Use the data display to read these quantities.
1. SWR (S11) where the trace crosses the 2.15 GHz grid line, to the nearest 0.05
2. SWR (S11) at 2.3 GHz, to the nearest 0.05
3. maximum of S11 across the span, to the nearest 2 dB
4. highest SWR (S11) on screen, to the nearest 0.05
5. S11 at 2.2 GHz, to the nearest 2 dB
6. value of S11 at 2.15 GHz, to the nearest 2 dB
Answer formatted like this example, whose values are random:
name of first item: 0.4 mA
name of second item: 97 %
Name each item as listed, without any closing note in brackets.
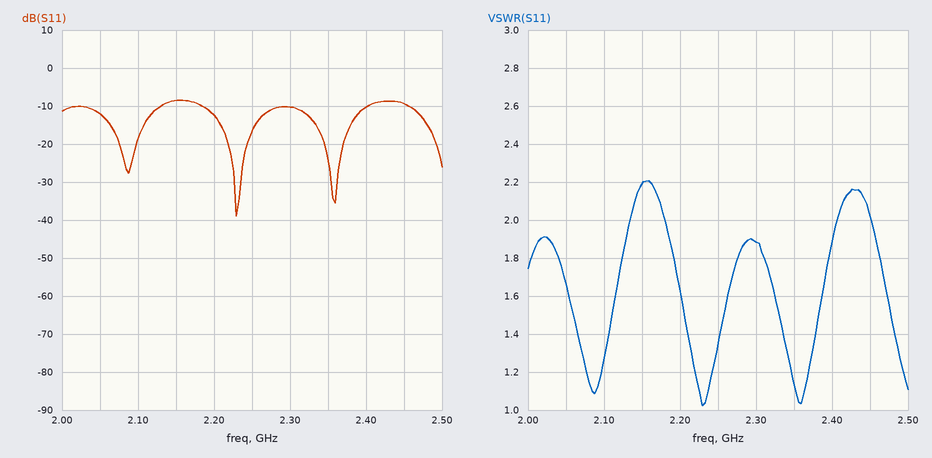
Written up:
SWR (S11) where the trace crosses the 2.15 GHz grid line, to the nearest 0.05: 2.20
SWR (S11) at 2.3 GHz, to the nearest 0.05: 1.90
maximum of S11 across the span, to the nearest 2 dB: -8 dB
highest SWR (S11) on screen, to the nearest 0.05: 2.20
S11 at 2.2 GHz, to the nearest 2 dB: -12 dB
value of S11 at 2.15 GHz, to the nearest 2 dB: -8 dB
